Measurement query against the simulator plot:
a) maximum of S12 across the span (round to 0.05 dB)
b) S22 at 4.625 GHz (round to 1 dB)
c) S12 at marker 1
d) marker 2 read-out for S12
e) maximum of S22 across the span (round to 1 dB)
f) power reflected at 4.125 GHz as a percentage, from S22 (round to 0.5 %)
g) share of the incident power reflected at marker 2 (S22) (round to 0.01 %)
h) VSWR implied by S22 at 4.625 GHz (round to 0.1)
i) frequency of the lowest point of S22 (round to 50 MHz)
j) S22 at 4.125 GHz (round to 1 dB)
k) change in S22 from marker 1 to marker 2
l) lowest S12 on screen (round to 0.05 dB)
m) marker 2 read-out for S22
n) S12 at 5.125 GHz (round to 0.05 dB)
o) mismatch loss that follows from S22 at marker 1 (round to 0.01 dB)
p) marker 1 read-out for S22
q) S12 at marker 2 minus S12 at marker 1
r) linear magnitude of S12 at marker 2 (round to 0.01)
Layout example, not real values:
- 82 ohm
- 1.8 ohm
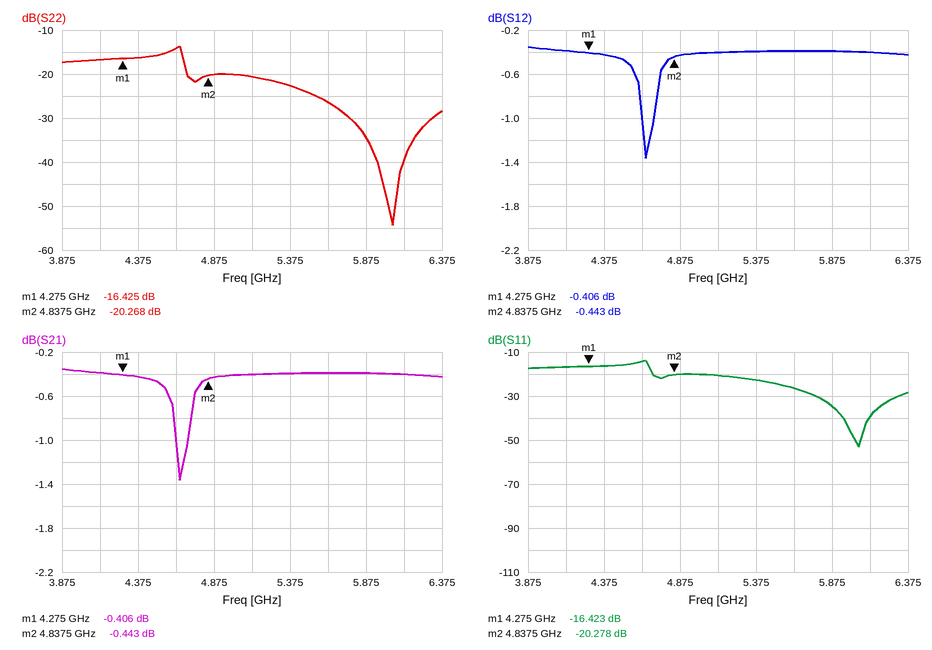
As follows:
- -0.35 dB
- -14 dB
- -0.406 dB
- -0.443 dB
- -14 dB
- 2.0 %
- 0.94 %
- 1.5
- 6.05 GHz
- -17 dB
- -3.843 dB
- -1.35 dB
- -20.268 dB
- -0.40 dB
- 0.10 dB
- -16.425 dB
- -0.037 dB
- 0.95
